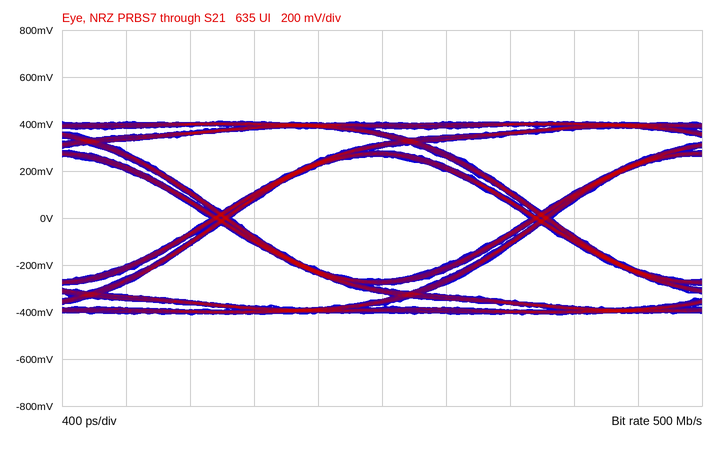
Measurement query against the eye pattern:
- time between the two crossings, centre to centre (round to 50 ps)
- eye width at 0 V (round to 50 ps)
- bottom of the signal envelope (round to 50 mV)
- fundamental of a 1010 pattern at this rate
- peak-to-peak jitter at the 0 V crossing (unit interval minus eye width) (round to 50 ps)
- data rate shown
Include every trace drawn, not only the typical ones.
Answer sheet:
2.00 ns
1.85 ns
-400 mV
250 MHz
150 ps
500 Mb/s
